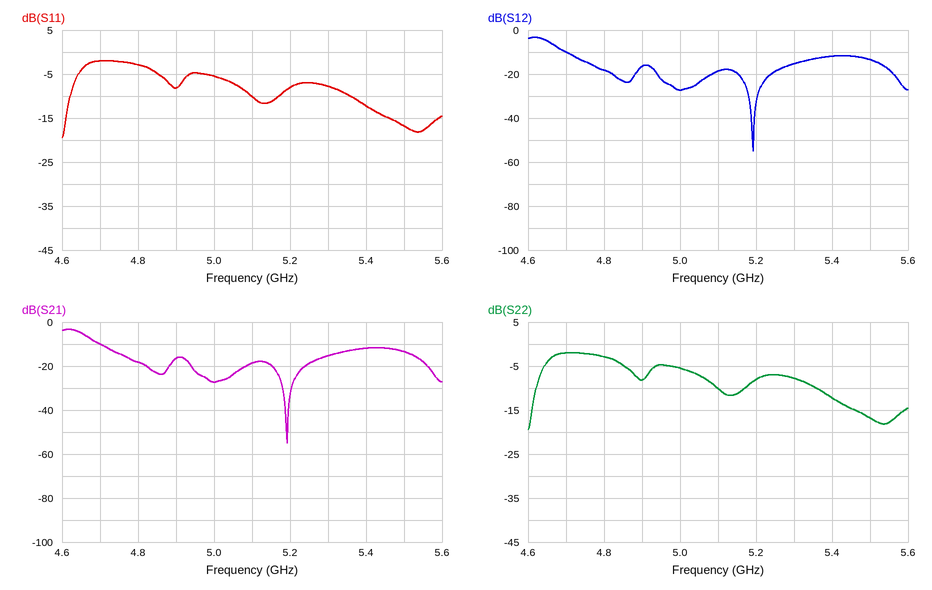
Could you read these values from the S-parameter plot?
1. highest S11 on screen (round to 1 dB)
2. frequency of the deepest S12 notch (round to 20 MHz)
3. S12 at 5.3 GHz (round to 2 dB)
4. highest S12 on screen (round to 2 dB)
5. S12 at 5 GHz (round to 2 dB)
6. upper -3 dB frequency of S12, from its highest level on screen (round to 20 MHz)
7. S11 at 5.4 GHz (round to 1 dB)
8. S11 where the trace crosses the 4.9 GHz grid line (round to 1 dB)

-2 dB
5.20 GHz
-16 dB
-4 dB
-28 dB
4.66 GHz
-12 dB
-8 dB
